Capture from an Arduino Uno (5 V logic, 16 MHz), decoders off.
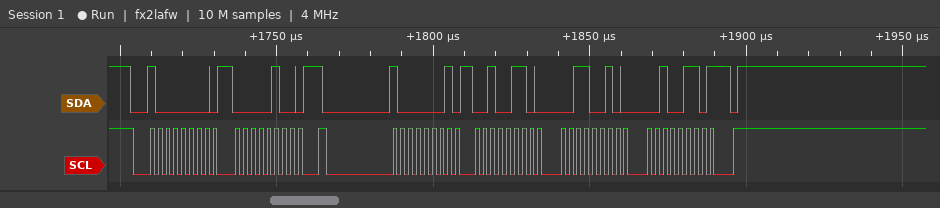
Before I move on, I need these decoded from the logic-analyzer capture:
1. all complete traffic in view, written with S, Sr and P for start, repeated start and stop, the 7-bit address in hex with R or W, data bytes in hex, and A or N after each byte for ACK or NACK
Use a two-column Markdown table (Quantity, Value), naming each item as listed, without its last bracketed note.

| Quantity | Value |
|---|---|
| all complete traffic in view, written with S, Sr and P for start, repeated start and stop, the 7-bit address in hex with R or W, data bytes in hex, and A or N after each byte for ACK or NACK | S 40W A 04 A Sr 40R A 26 A 32 A 26 N P |
